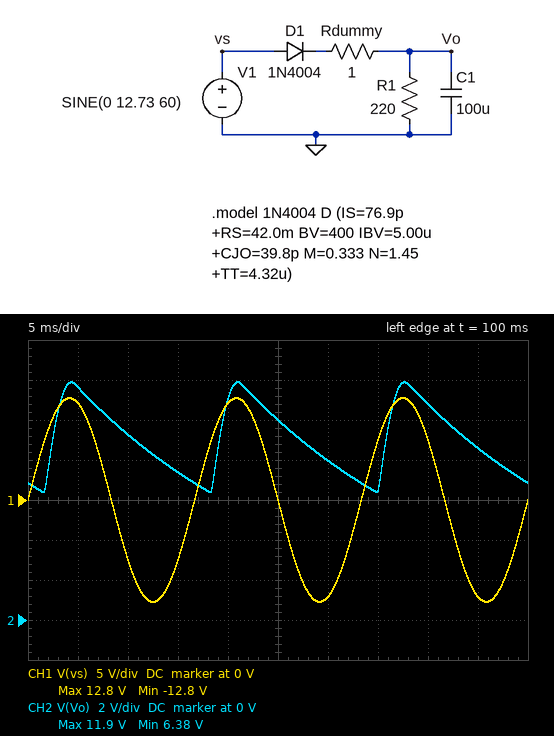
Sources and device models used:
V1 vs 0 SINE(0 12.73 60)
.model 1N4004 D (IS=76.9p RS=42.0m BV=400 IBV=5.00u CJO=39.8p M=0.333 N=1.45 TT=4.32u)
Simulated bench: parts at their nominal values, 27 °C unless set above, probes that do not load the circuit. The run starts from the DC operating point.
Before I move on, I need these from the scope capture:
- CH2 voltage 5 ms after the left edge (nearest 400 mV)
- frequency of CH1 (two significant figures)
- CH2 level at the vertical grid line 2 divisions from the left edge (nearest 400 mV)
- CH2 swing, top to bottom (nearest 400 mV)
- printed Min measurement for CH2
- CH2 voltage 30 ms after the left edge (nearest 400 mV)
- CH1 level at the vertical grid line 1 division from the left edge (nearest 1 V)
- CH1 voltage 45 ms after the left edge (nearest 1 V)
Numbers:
11.6 V
60 Hz
9.2 V
5.6 V
6.38 V
8.0 V
12 V
-12 V
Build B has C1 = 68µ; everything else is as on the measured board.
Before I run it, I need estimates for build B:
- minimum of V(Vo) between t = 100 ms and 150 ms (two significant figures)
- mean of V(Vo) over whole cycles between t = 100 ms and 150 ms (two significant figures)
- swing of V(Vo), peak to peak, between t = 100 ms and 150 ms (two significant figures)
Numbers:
4.9 V
8.2 V
7.0 V
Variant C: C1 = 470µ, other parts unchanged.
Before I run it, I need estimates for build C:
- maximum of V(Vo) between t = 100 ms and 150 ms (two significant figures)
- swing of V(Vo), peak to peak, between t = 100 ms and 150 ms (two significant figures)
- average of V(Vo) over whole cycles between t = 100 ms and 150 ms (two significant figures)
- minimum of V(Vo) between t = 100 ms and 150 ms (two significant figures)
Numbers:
12 V
1.5 V
11 V
10 V
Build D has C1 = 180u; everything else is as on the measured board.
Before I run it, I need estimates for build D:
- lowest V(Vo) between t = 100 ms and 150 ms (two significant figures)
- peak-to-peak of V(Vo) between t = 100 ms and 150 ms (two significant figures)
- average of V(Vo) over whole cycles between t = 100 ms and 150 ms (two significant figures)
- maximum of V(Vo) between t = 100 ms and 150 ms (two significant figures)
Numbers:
8.3 V
3.6 V
10 V
12 V
